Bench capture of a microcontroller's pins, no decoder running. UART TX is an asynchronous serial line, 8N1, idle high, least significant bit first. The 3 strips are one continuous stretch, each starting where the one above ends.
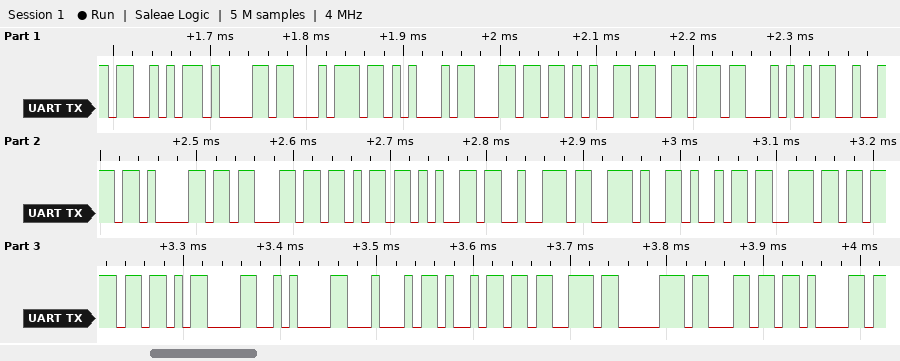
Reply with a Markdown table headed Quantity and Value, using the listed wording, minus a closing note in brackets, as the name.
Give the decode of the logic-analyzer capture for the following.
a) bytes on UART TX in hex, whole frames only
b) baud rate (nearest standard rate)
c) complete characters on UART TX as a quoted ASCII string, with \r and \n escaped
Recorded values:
| Quantity | Value |
|---|---|
| bytes on UART TX in hex, whole frames only | 0x53 0x61 0x74 0x45 0x6C 0x65 0x76 0x54 0x72 0x61 0x63 0x6B 0x65 0x72 0x2E 0x69 0x6E 0x6F 0x0D 0x0A 0x44 0x69 0x73 0x70 0x6C 0x61 |
| baud rate | 115200 baud |
| complete characters on UART TX as a quoted ASCII string, with \r and \n escaped | "SatElevTracker.ino\r\nDispla" |
